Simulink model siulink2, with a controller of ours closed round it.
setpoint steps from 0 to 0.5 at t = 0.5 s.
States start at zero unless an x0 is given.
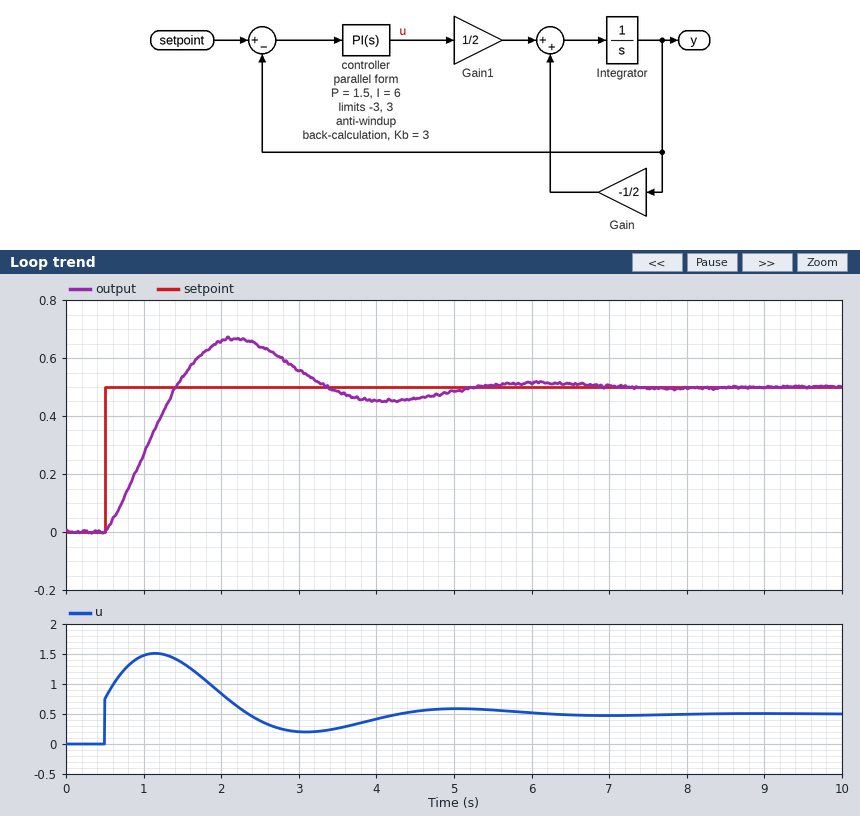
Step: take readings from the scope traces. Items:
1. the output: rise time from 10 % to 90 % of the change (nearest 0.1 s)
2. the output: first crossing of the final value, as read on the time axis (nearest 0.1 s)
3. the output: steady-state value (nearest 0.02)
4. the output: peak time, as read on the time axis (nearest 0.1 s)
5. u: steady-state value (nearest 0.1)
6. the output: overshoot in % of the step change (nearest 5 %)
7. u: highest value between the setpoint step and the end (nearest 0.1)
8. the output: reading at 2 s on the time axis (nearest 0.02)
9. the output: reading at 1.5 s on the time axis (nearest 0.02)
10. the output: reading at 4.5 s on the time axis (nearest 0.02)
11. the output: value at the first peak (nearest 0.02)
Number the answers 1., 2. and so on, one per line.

1. 0.7 s
2. 1.4 s
3. 0.50
4. 2.2 s
5. 0.5
6. 35 %
7. 1.5
8. 0.66
9. 0.54
10. 0.46
11. 0.66
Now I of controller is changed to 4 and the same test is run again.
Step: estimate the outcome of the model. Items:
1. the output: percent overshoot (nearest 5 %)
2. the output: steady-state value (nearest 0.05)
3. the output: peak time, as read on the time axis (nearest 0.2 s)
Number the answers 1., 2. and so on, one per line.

1. 25 %
2. 0.50
3. 2.6 s
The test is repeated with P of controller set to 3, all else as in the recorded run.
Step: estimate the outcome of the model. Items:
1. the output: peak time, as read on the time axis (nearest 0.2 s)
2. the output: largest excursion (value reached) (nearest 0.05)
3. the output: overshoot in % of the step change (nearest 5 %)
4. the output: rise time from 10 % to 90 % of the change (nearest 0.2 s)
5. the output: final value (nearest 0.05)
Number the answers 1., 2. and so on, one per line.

1. 2.0 s
2. 0.60
3. 20 %
4. 0.6 s
5. 0.50
